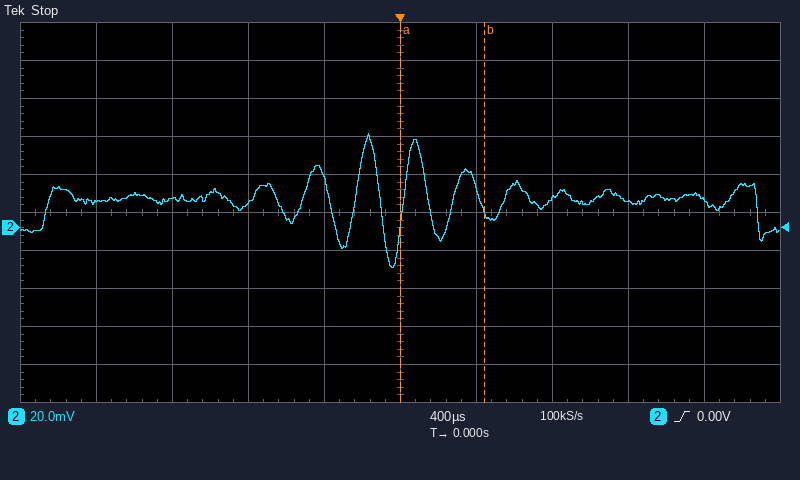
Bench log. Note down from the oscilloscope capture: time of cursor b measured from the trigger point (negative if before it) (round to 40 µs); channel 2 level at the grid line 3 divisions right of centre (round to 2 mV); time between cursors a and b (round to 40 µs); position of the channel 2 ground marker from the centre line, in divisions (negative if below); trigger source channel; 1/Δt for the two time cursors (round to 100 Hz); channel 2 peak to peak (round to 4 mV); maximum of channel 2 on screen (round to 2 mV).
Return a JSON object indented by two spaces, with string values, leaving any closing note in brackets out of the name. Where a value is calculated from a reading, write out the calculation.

{
  "time of cursor b measured from the trigger point (negative if before it)": "+440 µs",
  "channel 2 level at the grid line 3 divisions right of centre": "14 mV",
  "time between cursors a and b": "440 µs",
  "position of the channel 2 ground marker from the centre line, in divisions": "-0.4 div",
  "trigger source channel": "channel 2",
  "1/Δt for the two time cursors": "1 / 440 µs ≈ 2.3 kHz",
  "channel 2 peak to peak": "72 mV",
  "maximum of channel 2 on screen": "50 mV"
}
